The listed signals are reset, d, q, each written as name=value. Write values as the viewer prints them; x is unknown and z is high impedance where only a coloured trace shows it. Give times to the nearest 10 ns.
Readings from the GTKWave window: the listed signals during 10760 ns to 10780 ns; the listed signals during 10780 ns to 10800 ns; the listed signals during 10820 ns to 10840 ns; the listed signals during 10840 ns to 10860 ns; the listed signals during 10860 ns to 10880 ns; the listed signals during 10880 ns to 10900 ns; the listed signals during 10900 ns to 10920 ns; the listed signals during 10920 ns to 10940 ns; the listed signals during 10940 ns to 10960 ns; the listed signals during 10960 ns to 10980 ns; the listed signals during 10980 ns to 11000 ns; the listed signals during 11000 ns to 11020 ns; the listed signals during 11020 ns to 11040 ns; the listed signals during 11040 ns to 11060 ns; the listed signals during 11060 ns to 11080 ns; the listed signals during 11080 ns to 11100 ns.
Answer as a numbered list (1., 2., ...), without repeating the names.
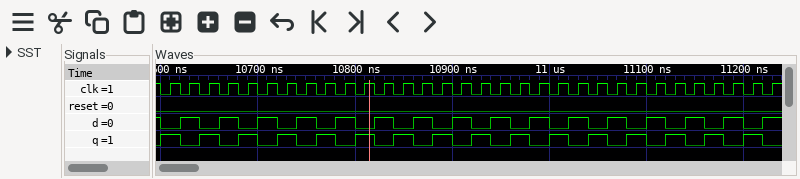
1. reset=0, d=0, q=1
2. reset=0, d=1, q=0
3. reset=0, d=1, q=0
4. reset=0, d=0, q=1
5. reset=0, d=1, q=0
6. reset=0, d=0, q=1
7. reset=0, d=1, q=0
8. reset=0, d=0, q=1
9. reset=0, d=1, q=0
10. reset=0, d=0, q=1
11. reset=0, d=1, q=0
12. reset=0, d=0, q=1
13. reset=0, d=1, q=0
14. reset=0, d=0, q=1
15. reset=0, d=1, q=0
16. reset=0, d=0, q=1
